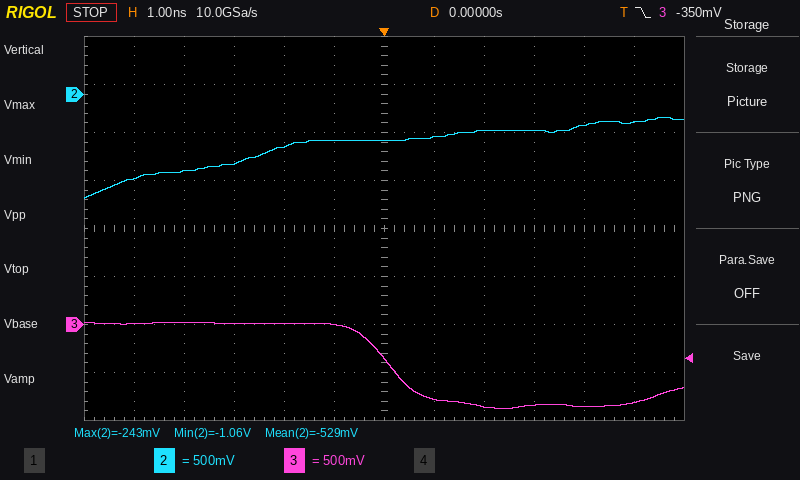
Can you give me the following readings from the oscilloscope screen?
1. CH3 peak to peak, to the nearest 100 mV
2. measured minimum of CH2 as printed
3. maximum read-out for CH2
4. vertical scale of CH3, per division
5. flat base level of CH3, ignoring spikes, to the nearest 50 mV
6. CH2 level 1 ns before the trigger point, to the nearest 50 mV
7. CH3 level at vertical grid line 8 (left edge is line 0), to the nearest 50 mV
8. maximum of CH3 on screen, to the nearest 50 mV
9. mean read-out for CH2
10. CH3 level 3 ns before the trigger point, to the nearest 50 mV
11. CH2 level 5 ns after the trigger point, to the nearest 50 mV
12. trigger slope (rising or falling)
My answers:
900 mV
-1.06 V
-243 mV
500 mV
-850 mV
-500 mV
-850 mV
0 mV
-529 mV
0 mV
-300 mV
falling
